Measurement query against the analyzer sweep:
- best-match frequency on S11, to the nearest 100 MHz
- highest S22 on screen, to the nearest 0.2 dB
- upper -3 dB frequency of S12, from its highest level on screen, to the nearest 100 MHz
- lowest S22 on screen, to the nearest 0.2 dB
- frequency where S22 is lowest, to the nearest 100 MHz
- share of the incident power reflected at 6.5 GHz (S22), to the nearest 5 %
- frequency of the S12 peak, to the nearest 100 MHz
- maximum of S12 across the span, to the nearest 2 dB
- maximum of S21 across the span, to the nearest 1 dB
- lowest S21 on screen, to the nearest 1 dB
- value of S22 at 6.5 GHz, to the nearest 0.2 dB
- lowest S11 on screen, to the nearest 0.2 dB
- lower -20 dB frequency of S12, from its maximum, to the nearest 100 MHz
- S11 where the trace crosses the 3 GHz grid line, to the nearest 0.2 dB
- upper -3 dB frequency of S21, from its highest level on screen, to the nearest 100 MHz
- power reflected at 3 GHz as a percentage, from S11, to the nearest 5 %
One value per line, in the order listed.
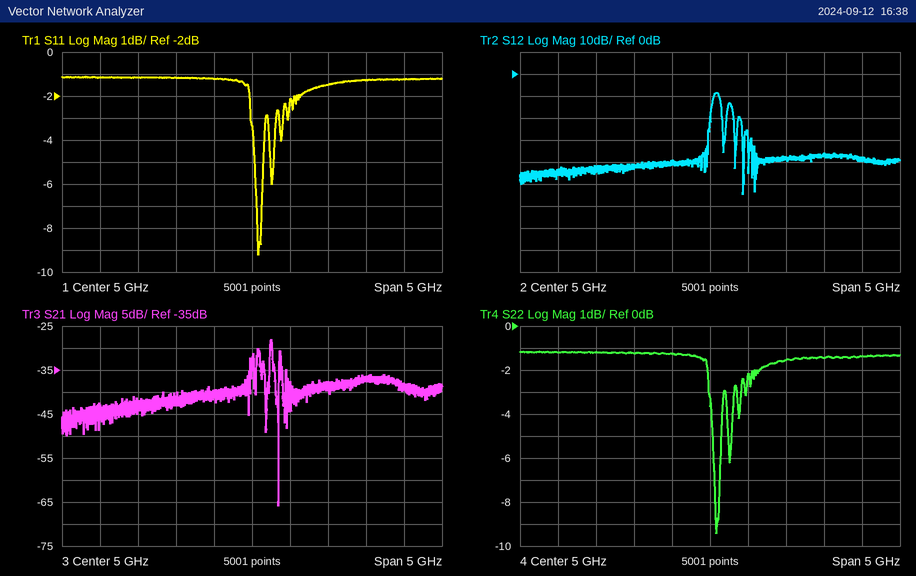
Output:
5.1 GHz
-1.2 dB
5.1 GHz
-9.4 dB
5.1 GHz
70 %
5.1 GHz
-8 dB
-28 dB
-66 dB
-1.4 dB
-9.2 dB
5.0 GHz
-1.2 dB
5.3 GHz
75 %
